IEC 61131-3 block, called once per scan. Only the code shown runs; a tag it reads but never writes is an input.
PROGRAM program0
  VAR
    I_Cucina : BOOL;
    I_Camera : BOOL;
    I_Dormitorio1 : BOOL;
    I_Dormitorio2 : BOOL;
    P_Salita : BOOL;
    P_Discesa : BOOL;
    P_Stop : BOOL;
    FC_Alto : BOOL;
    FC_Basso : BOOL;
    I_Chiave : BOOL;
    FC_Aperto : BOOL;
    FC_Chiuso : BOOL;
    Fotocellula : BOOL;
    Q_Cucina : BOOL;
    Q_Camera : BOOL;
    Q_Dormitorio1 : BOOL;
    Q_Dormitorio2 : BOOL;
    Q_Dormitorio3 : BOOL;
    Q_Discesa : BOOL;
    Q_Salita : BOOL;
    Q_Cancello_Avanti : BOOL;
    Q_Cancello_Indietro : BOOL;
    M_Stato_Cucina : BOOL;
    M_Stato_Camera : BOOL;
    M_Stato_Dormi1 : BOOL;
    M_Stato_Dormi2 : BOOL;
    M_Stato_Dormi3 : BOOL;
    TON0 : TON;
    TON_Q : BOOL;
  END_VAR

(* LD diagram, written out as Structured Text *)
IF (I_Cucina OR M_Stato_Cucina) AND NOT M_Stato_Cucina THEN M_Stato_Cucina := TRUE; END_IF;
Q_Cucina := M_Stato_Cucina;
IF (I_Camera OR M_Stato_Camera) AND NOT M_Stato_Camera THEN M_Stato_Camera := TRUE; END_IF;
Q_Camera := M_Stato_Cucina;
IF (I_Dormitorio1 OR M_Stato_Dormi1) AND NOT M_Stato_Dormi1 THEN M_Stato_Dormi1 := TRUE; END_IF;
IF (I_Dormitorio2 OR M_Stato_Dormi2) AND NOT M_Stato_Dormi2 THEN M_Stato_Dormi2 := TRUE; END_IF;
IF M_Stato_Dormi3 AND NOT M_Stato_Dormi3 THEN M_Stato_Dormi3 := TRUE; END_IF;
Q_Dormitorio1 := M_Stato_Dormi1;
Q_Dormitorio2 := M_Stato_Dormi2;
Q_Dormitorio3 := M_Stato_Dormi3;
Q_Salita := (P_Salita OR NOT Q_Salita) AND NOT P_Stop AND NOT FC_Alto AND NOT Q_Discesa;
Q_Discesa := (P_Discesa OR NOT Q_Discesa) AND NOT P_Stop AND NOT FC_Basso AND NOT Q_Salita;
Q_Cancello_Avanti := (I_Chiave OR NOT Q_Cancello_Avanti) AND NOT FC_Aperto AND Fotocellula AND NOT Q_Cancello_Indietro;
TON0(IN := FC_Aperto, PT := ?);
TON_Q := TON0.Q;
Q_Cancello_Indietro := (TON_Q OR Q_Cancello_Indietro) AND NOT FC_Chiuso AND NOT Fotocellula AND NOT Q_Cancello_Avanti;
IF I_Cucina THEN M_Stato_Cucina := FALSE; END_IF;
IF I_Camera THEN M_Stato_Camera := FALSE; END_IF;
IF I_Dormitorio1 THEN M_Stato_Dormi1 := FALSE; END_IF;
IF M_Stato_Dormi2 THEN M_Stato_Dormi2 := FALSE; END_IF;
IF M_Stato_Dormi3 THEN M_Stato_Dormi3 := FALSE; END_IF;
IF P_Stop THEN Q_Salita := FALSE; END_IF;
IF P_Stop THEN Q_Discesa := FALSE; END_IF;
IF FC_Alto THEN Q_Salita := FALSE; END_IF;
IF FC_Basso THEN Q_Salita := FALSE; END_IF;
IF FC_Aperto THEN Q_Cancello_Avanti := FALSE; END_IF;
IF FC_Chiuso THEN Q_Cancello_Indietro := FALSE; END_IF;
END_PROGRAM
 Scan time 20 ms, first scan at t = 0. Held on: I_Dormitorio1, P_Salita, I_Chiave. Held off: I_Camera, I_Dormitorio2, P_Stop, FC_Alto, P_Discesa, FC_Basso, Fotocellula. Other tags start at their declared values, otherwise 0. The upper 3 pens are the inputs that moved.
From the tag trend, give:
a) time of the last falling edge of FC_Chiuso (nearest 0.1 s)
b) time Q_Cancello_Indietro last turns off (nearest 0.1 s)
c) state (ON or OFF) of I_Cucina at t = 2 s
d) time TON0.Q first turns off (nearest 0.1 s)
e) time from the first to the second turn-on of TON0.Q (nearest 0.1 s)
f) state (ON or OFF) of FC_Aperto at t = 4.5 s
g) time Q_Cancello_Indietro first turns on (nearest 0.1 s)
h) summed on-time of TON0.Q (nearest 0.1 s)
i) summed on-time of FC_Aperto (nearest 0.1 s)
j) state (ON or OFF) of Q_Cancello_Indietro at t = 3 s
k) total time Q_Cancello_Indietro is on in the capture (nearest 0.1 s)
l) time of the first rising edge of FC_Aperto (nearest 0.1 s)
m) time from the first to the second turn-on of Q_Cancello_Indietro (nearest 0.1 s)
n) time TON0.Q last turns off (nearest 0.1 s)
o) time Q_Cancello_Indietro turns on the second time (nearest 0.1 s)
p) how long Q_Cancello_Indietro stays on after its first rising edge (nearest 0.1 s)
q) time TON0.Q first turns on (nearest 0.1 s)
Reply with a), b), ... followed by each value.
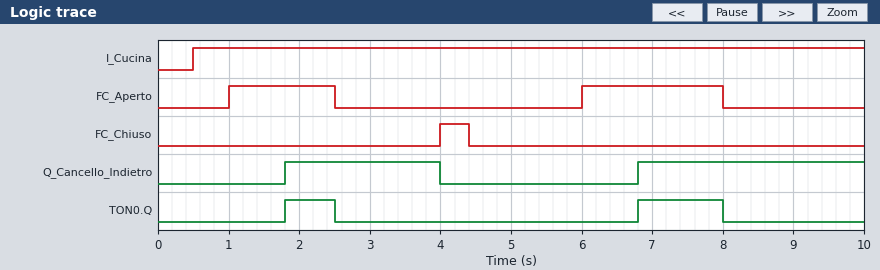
a) 4.4 s
b) 4.0 s
c) ON
d) 2.5 s
e) 5.0 s
f) OFF
g) 1.8 s
h) 1.9 s
i) 3.5 s
j) ON
k) 5.4 s
l) 1.0 s
m) 5.0 s
n) 8.0 s
o) 6.8 s
p) 2.2 s
q) 1.8 s
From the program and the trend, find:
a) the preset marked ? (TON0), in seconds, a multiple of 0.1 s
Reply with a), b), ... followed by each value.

a) 0.8 s
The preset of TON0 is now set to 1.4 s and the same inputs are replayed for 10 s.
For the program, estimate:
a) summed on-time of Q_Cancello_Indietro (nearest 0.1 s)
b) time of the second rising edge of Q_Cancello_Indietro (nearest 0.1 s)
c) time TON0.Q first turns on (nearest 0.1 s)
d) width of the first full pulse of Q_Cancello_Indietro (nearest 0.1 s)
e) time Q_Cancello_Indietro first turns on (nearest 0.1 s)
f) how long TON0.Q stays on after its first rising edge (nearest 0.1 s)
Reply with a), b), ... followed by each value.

a) 4.2 s
b) 7.4 s
c) 2.4 s
d) 1.6 s
e) 2.4 s
f) 0.1 s
